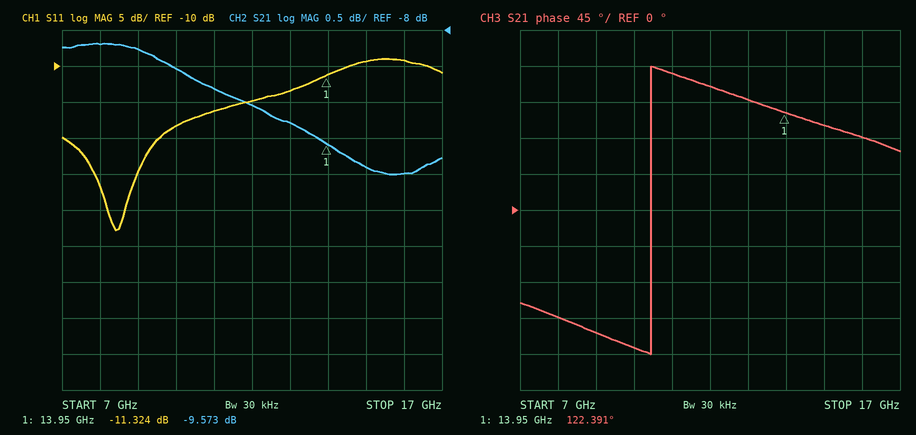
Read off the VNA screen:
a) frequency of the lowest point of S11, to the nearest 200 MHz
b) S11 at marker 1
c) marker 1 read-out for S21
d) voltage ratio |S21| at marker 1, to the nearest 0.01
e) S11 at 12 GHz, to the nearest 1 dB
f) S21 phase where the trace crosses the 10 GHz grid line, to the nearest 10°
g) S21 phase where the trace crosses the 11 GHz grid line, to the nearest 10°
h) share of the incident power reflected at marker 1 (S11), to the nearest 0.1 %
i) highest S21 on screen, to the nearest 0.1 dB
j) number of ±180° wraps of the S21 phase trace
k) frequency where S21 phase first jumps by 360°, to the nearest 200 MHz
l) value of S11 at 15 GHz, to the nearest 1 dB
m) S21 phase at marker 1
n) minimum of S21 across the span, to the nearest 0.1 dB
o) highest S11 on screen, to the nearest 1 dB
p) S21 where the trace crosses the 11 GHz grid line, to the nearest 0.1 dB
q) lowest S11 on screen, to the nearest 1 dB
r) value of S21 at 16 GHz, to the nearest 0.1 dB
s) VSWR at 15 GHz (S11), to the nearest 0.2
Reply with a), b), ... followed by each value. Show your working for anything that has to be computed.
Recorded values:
a) 8.4 GHz
b) -11.324 dB
c) -9.573 dB
d) 10^(-9.573/20) ≈ 0.33
e) -15 dB
f) -170°
g) 170°
h) 10^(-11.324/10) ≈ 7.4 %
i) -8.2 dB
j) 1
k) 10.4 GHz
l) -9 dB
m) 122.391°
n) -10.0 dB
o) -9 dB
p) -8.8 dB
q) -33 dB
r) -10.0 dB
s) |Γ| = 10^(-9/20) = 0.3548; VSWR = (1 + 0.3548)/(1 − 0.3548) ≈ 2.10, so 2.0 to the nearest 0.2
